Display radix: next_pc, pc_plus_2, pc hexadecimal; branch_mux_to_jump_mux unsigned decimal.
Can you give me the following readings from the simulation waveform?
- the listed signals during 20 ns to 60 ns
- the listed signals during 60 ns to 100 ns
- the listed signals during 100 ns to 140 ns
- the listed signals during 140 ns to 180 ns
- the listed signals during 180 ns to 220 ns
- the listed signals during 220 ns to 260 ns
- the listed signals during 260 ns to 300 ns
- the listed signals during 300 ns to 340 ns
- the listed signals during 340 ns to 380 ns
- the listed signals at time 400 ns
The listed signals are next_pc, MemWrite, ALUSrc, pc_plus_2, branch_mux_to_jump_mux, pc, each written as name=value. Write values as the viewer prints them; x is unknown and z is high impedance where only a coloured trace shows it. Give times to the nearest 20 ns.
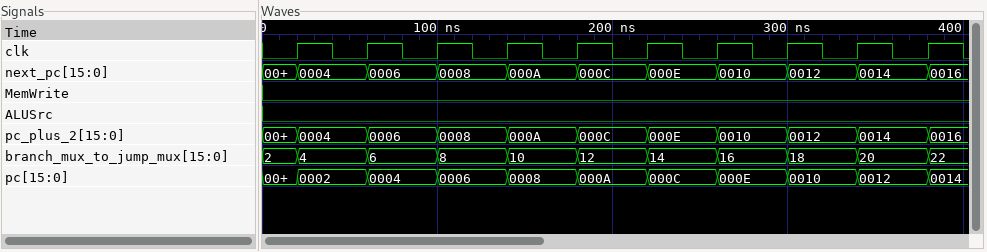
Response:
next_pc=0004, MemWrite=0, ALUSrc=0, pc_plus_2=0004, branch_mux_to_jump_mux=4, pc=0002
next_pc=0006, MemWrite=0, ALUSrc=0, pc_plus_2=0006, branch_mux_to_jump_mux=6, pc=0004
next_pc=0008, MemWrite=0, ALUSrc=0, pc_plus_2=0008, branch_mux_to_jump_mux=8, pc=0006
next_pc=000A, MemWrite=0, ALUSrc=0, pc_plus_2=000A, branch_mux_to_jump_mux=10, pc=0008
next_pc=000C, MemWrite=0, ALUSrc=0, pc_plus_2=000C, branch_mux_to_jump_mux=12, pc=000A
next_pc=000E, MemWrite=0, ALUSrc=0, pc_plus_2=000E, branch_mux_to_jump_mux=14, pc=000C
next_pc=0010, MemWrite=0, ALUSrc=0, pc_plus_2=0010, branch_mux_to_jump_mux=16, pc=000E
next_pc=0012, MemWrite=0, ALUSrc=0, pc_plus_2=0012, branch_mux_to_jump_mux=18, pc=0010
next_pc=0014, MemWrite=0, ALUSrc=0, pc_plus_2=0014, branch_mux_to_jump_mux=20, pc=0012
next_pc=0016, MemWrite=0, ALUSrc=0, pc_plus_2=0016, branch_mux_to_jump_mux=22, pc=0014
